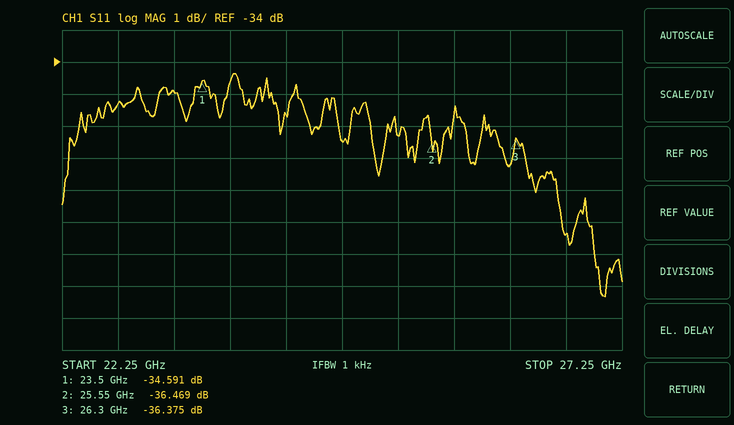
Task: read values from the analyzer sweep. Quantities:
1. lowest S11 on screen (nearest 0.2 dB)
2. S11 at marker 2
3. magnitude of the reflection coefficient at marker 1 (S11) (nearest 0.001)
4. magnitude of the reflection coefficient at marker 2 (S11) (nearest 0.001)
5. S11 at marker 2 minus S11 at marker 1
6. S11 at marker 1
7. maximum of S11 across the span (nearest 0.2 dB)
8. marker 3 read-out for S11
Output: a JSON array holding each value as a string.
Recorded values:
["-41.4 dB", "-36.469 dB", "0.019", "0.015", "-1.878 dB", "-34.591 dB", "-34.4 dB", "-36.375 dB"]
